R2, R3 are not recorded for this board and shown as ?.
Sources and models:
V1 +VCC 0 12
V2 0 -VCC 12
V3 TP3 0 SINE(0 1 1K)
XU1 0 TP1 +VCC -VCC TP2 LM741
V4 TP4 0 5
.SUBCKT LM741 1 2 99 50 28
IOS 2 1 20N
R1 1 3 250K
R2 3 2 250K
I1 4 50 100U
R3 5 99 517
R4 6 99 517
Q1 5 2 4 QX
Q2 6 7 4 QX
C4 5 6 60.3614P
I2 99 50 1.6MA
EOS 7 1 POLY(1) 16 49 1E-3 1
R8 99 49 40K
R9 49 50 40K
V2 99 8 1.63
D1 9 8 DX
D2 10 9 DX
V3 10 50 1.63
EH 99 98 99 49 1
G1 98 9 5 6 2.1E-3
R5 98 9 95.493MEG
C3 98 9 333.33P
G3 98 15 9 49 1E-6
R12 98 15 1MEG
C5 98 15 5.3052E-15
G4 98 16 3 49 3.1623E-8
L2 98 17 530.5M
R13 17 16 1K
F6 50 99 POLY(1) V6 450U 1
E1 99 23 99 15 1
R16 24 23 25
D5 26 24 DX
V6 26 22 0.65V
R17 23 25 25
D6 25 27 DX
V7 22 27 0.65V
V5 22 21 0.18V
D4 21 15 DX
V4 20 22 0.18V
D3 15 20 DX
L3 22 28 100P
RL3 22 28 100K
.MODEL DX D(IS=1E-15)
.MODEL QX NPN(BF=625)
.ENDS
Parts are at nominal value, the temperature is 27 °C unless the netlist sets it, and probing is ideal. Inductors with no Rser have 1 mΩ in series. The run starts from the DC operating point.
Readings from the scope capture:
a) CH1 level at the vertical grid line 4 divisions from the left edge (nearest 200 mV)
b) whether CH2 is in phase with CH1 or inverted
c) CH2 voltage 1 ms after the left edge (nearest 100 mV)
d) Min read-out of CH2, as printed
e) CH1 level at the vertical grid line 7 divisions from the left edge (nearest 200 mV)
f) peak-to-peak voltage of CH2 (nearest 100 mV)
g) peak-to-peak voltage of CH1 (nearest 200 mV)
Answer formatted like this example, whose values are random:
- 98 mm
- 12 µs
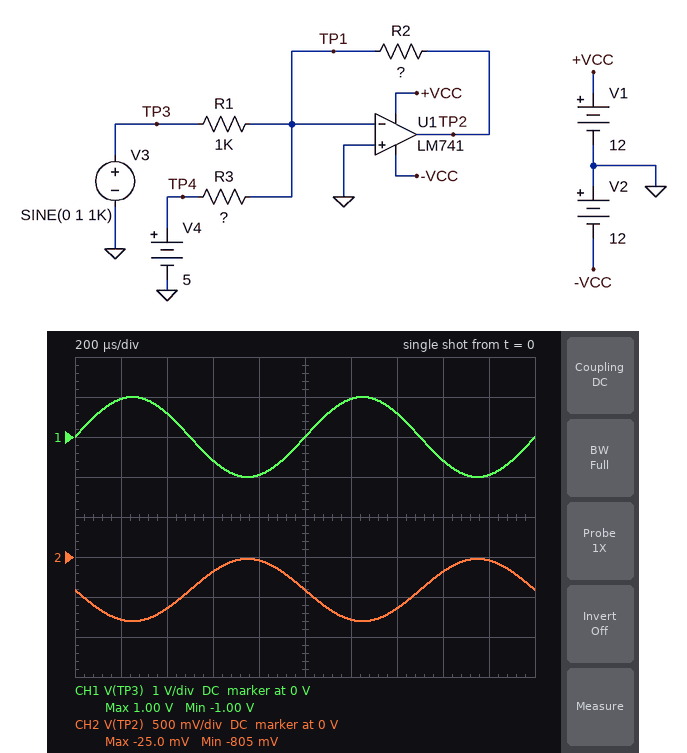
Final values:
- -1.0 V
- inverted
- -400 mV
- -805 mV
- 600 mV
- 800 mV
- 2.0 V
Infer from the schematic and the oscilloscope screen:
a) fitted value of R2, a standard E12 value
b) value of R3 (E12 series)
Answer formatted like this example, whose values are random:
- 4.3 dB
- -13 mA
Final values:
- 390 Ω
- 4.7 kΩ
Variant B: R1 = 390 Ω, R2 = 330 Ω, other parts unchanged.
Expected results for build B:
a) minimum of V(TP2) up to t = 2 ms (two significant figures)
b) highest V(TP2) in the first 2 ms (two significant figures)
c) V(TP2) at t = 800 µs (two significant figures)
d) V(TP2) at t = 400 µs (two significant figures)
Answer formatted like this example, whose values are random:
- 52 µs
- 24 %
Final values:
- -1.2 V
- 500 mV
- 460 mV
- -850 mV
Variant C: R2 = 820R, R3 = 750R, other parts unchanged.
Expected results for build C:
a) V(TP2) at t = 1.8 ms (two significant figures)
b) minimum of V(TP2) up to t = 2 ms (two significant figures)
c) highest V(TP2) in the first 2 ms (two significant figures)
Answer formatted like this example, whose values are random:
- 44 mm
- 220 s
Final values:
- -4.7 V
- -6.3 V
- -4.6 V
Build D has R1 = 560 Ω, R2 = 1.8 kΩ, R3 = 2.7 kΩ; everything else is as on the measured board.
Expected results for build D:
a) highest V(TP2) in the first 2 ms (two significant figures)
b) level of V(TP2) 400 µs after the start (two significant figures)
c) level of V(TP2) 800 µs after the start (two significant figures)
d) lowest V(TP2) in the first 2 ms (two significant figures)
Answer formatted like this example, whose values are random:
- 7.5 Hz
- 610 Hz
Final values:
- -110 mV
- -5.2 V
- -270 mV
- -6.5 V
